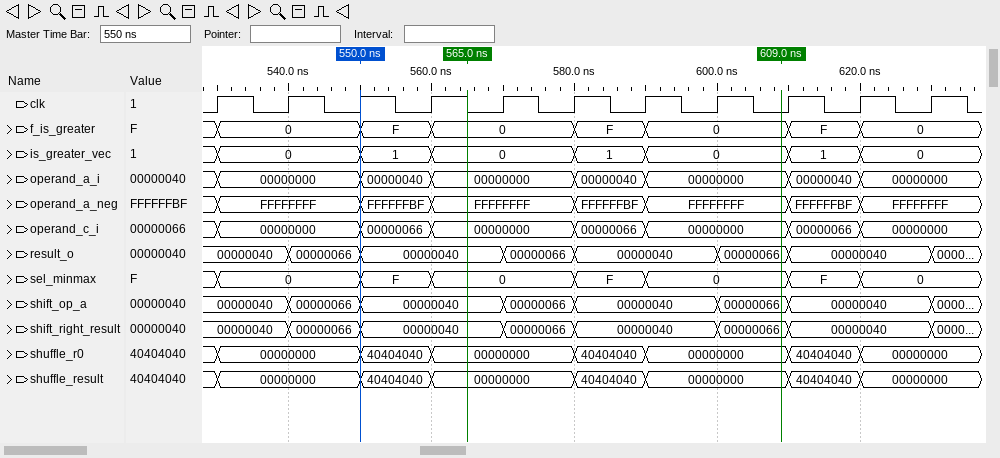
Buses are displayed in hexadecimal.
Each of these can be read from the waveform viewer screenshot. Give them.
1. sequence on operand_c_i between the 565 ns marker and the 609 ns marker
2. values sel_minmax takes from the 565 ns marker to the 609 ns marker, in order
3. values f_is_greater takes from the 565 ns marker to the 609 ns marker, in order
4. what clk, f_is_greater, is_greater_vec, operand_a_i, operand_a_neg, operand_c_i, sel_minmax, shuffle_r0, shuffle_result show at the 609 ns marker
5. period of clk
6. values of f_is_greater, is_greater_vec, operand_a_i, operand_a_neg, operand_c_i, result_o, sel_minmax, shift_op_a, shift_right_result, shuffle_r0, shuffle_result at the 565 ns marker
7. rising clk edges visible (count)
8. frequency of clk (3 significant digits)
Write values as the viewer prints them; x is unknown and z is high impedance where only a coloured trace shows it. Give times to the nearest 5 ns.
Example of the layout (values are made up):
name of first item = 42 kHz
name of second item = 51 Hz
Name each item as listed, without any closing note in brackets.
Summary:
sequence on operand_c_i between the 565 ns marker and the 609 ns marker = 00000000, 00000066, 00000000
values sel_minmax takes from the 565 ns marker to the 609 ns marker, in order = 0, F, 0
values f_is_greater takes from the 565 ns marker to the 609 ns marker, in order = 0, F, 0
what clk, f_is_greater, is_greater_vec, operand_a_i, operand_a_neg, operand_c_i, sel_minmax, shuffle_r0, shuffle_result show at the 609 ns marker = clk=0, f_is_greater=0, is_greater_vec=0, operand_a_i=00000000, operand_a_neg=FFFFFFFF, operand_c_i=00000000, sel_minmax=0, shuffle_r0=00000000, shuffle_result=00000000
period of clk = 10 ns
values of f_is_greater, is_greater_vec, operand_a_i, operand_a_neg, operand_c_i, result_o, sel_minmax, shift_op_a, shift_right_result, shuffle_r0, shuffle_result at the 565 ns marker = f_is_greater=0, is_greater_vec=0, operand_a_i=00000000, operand_a_neg=FFFFFFFF, operand_c_i=00000000, result_o=00000040, sel_minmax=0, shift_op_a=00000040, shift_right_result=00000040, shuffle_r0=00000000, shuffle_result=00000000
rising clk edges visible = 11
frequency of clk = 100 MHz
